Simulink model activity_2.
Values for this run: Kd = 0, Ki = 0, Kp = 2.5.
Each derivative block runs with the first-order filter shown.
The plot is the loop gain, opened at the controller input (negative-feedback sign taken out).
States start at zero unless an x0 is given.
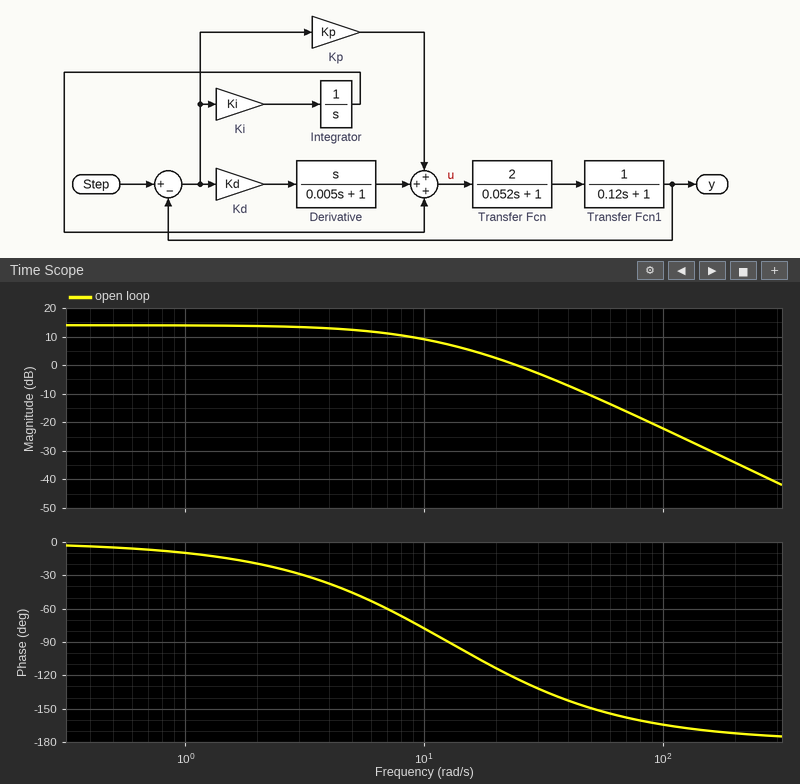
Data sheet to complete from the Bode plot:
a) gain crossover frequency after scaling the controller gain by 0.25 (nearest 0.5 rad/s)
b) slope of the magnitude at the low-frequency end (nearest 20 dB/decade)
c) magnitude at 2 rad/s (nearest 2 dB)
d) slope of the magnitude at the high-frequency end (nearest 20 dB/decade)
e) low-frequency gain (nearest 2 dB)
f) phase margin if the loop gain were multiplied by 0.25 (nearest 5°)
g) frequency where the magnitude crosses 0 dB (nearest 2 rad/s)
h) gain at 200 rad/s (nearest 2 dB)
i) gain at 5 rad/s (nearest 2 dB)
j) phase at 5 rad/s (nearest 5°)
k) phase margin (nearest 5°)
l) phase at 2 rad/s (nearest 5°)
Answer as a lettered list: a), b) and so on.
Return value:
a) 5.5 rad/s
b) 0 dB/decade
c) 14 dB
d) -40 dB/decade
e) 14 dB
f) 130°
g) 24 rad/s
h) -34 dB
i) 12 dB
j) -45°
k) 55°
l) -20°
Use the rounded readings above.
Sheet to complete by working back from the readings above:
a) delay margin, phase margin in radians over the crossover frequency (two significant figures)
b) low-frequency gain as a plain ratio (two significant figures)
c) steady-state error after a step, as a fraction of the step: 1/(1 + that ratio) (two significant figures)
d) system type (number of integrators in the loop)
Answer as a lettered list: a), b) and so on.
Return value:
a) 0.040 s
b) 5.0
c) 0.17
d) 0
